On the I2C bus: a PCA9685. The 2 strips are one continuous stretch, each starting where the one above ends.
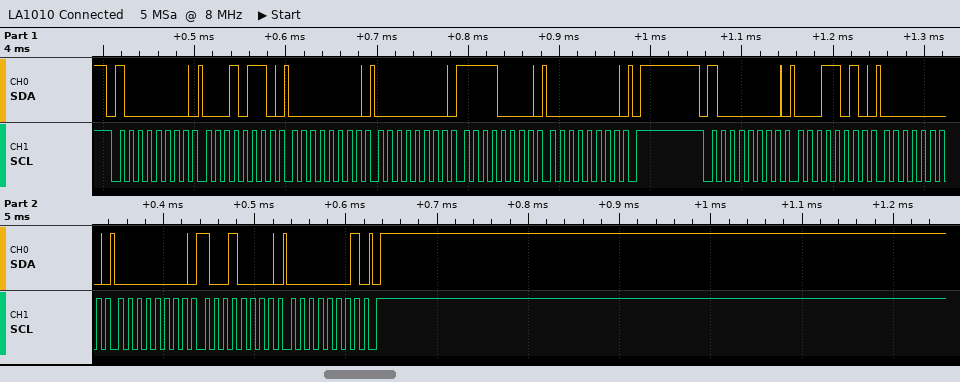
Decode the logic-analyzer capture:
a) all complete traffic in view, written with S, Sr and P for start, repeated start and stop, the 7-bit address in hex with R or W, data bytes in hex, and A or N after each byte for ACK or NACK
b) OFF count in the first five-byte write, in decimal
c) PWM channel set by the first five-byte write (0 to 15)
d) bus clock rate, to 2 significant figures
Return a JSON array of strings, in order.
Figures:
["S 40W A 16 A 00 A 00 A F0 A 00 A P S 40W A 1A A 00 A 00 A 90 A 01 A P", "240", "4", "100 kHz"]
